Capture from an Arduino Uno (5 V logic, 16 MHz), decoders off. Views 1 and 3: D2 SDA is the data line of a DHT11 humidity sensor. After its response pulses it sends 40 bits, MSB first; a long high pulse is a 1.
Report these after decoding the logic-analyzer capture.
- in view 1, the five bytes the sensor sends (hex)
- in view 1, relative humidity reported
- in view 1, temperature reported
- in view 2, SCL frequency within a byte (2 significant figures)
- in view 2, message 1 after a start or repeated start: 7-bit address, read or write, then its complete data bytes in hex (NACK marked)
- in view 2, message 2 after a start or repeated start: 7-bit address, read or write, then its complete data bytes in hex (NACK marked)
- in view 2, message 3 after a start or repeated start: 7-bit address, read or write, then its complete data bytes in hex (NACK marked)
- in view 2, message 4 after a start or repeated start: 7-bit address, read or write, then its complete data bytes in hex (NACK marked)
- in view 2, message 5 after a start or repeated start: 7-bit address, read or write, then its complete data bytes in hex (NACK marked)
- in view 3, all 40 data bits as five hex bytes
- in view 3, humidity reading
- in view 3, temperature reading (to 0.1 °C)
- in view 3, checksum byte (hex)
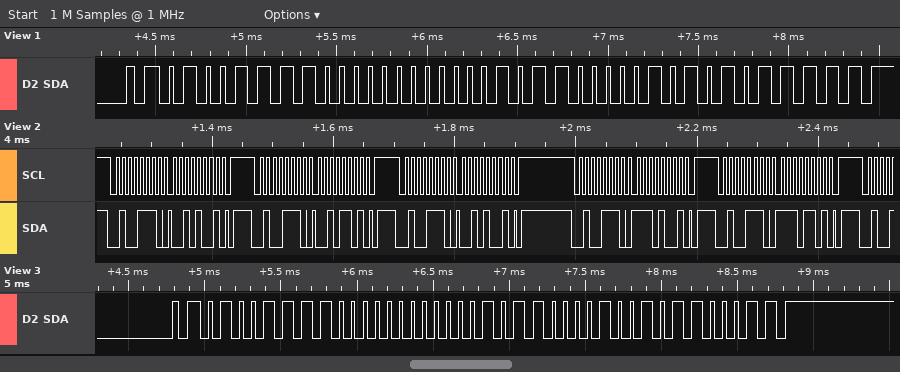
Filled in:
4F 00 0B 05 5F
79 %
11.5 °C
100 kHz
0x27 write: 29
0x27 write: 2D
0x27 write: 29
0x27 write: E9
0x27 write: ED
4F 00 0B 09 63
79 %
11.9 °C
0x63
